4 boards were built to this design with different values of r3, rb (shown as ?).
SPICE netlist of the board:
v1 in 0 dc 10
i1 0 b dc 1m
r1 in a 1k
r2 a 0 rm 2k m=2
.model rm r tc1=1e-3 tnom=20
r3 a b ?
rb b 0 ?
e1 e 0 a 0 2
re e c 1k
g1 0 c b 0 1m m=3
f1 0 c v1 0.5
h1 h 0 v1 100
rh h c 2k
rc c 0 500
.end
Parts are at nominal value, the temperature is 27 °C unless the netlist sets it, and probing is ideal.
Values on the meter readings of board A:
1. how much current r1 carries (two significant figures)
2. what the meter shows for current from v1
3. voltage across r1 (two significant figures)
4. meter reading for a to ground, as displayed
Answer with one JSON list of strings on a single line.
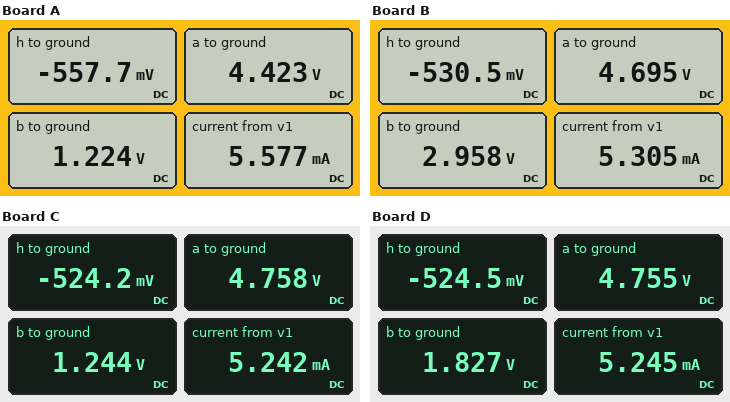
["5.6 mA", "5.577 mA", "5.6 V", "4.423 V"]
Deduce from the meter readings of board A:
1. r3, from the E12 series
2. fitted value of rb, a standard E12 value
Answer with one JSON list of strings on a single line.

["2.7 kΩ", "560 Ω"]
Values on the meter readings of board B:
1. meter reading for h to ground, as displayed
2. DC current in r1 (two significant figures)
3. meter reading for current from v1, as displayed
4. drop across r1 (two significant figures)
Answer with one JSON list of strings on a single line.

["-530.5 mV", "5.3 mA", "5.305 mA", "5.3 V"]
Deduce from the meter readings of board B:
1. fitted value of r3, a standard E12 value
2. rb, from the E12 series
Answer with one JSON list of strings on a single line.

["2.7 kΩ", "1.8 kΩ"]
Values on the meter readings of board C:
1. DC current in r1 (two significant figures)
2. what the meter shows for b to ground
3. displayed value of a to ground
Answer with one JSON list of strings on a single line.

["5.2 mA", "1.244 V", "4.758 V"]
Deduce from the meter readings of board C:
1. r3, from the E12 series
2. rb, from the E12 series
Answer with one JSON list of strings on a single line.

["6.8 kΩ", "820 Ω"]
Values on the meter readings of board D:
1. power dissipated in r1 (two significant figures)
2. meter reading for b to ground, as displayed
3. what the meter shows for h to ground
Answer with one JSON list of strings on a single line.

["28 mW", "1.827 V", "-524.5 mV"]
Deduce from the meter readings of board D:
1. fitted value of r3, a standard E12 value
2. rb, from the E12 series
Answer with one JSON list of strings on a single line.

["5.6 kΩ", "1.2 kΩ"]
